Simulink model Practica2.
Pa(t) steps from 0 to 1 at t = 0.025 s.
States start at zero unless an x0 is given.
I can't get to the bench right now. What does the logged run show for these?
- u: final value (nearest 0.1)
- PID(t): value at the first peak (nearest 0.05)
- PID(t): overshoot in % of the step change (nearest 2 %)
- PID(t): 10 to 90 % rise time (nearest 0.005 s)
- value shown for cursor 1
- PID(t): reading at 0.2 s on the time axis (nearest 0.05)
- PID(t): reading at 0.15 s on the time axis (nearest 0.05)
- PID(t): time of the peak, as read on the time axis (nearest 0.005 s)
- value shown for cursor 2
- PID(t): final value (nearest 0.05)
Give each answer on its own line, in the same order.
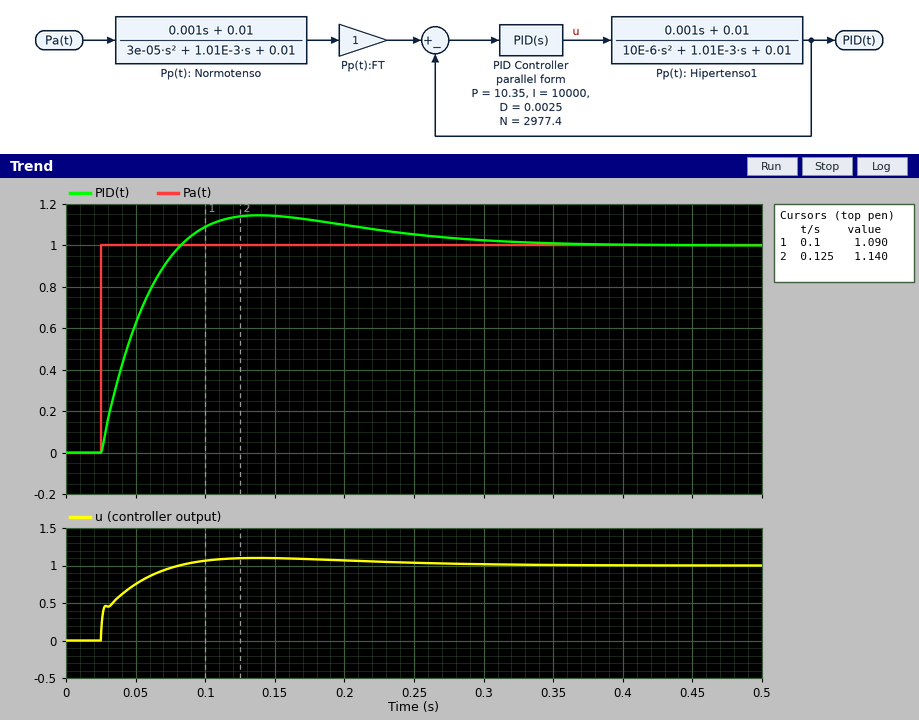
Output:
1.0
1.15
14 %
0.040 s
1.090
1.10
1.15
0.140 s
1.140
1.00
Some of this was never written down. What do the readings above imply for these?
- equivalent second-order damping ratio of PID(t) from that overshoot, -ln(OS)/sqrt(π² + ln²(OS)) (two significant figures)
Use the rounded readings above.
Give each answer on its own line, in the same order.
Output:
0.53
